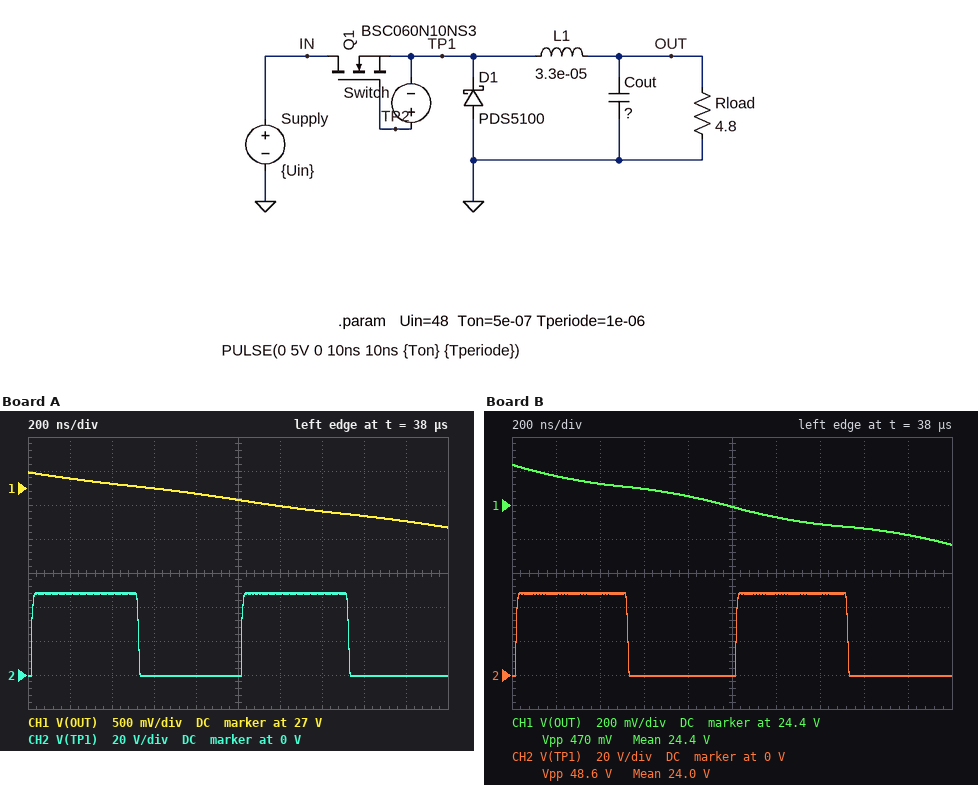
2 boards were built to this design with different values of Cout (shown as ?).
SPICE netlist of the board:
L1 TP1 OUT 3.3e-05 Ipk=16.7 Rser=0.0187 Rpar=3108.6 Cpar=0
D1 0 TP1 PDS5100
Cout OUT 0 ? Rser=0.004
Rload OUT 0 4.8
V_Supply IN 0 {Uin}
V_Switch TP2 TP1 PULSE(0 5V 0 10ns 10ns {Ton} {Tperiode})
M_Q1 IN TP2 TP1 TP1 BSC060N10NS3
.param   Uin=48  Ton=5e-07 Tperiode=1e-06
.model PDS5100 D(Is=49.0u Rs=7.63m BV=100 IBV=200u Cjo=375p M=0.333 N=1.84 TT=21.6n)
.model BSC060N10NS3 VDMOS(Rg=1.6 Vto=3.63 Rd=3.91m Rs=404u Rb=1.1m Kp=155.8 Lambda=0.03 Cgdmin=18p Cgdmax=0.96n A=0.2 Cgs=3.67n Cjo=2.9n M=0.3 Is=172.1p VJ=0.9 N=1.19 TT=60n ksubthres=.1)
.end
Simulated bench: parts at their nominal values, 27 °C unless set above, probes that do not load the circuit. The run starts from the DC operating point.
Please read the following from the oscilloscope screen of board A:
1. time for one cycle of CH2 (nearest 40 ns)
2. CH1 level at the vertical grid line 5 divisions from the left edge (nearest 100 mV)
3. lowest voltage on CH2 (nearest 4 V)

1.00 µs
26.8 V
0 V
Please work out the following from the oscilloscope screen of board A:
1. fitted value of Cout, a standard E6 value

2.2 µF
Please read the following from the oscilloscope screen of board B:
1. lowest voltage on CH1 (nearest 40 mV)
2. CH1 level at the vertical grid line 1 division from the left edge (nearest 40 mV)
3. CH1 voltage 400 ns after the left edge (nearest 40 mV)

24.16 V
24.56 V
24.52 V
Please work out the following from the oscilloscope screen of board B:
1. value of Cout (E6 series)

1.5 µF
